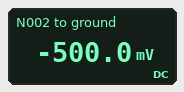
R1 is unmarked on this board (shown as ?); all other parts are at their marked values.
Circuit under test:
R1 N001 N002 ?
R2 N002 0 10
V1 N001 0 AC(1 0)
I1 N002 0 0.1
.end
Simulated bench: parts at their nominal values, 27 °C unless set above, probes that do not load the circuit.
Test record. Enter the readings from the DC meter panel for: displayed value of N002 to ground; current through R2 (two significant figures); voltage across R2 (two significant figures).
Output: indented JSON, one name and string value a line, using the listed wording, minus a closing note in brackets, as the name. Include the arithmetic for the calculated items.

{
  "displayed value of N002 to ground": "-500.0 mV",
  "current through R2": "(0 V - (-500 mV)) / 10 Ω = 50 mA",
  "voltage across R2": "0 V - (-500 mV) = 500 mV"
}
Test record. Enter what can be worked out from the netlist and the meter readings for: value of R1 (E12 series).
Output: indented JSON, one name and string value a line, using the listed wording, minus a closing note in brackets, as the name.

{
  "value of R1": "10 Ω"
}
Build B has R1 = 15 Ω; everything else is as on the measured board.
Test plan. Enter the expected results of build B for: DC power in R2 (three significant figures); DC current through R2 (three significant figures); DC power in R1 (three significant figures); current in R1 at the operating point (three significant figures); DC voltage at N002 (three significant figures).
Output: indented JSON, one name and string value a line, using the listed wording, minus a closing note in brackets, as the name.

{
  "DC power in R2": "36.0 mW",
  "DC current through R2": "60.0 mA",
  "DC power in R1": "24.0 mW",
  "current in R1 at the operating point": "40.0 mA",
  "DC voltage at N002": "-600 mV"
}
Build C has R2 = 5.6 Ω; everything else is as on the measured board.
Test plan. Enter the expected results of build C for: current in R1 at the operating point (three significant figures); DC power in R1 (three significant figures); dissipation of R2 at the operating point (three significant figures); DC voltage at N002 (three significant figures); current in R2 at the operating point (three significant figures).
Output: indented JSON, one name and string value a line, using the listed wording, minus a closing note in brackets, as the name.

{
  "current in R1 at the operating point": "35.9 mA",
  "DC power in R1": "12.9 mW",
  "dissipation of R2 at the operating point": "23.0 mW",
  "DC voltage at N002": "-359 mV",
  "current in R2 at the operating point": "64.1 mA"
}
